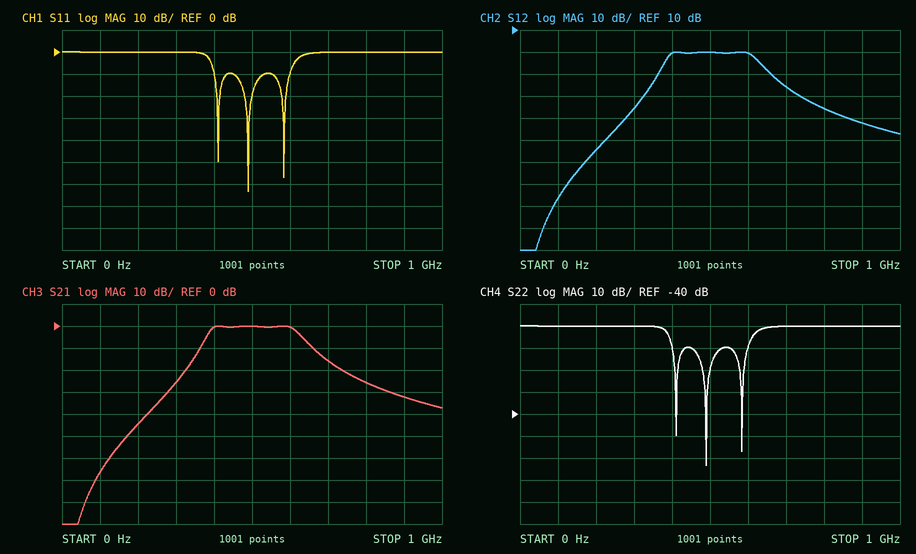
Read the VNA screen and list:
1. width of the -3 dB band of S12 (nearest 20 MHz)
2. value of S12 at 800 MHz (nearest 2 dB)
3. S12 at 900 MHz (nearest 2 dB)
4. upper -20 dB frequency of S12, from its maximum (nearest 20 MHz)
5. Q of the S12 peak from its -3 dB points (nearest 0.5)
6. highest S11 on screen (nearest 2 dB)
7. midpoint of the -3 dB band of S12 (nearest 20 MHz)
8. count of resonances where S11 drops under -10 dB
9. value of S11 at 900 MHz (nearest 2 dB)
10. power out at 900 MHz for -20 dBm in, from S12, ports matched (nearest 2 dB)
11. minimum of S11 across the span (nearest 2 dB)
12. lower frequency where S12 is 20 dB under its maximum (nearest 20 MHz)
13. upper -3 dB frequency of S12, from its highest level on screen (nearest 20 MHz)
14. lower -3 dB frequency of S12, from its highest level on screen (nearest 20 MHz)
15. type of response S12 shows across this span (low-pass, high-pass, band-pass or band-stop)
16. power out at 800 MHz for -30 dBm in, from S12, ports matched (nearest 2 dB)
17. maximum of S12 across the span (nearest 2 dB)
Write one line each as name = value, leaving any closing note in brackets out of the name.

width of the -3 dB band of S12 = 240 MHz
value of S12 at 800 MHz = -26 dB
S12 at 900 MHz = -32 dB
upper -20 dB frequency of S12, from its maximum = 740 MHz
Q of the S12 peak from its -3 dB points = 2.0
highest S11 on screen = 0 dB
midpoint of the -3 dB band of S12 = 500 MHz
count of resonances where S11 drops under -10 dB = 3
value of S11 at 900 MHz = 0 dB
power out at 900 MHz for -20 dBm in, from S12, ports matched = -52 dBm
minimum of S11 across the span = -64 dB
lower frequency where S12 is 20 dB under its maximum = 320 MHz
upper -3 dB frequency of S12, from its highest level on screen = 620 MHz
lower -3 dB frequency of S12, from its highest level on screen = 380 MHz
type of response S12 shows across this span = band-pass
power out at 800 MHz for -30 dBm in, from S12, ports matched = -56 dBm
maximum of S12 across the span = 0 dB
